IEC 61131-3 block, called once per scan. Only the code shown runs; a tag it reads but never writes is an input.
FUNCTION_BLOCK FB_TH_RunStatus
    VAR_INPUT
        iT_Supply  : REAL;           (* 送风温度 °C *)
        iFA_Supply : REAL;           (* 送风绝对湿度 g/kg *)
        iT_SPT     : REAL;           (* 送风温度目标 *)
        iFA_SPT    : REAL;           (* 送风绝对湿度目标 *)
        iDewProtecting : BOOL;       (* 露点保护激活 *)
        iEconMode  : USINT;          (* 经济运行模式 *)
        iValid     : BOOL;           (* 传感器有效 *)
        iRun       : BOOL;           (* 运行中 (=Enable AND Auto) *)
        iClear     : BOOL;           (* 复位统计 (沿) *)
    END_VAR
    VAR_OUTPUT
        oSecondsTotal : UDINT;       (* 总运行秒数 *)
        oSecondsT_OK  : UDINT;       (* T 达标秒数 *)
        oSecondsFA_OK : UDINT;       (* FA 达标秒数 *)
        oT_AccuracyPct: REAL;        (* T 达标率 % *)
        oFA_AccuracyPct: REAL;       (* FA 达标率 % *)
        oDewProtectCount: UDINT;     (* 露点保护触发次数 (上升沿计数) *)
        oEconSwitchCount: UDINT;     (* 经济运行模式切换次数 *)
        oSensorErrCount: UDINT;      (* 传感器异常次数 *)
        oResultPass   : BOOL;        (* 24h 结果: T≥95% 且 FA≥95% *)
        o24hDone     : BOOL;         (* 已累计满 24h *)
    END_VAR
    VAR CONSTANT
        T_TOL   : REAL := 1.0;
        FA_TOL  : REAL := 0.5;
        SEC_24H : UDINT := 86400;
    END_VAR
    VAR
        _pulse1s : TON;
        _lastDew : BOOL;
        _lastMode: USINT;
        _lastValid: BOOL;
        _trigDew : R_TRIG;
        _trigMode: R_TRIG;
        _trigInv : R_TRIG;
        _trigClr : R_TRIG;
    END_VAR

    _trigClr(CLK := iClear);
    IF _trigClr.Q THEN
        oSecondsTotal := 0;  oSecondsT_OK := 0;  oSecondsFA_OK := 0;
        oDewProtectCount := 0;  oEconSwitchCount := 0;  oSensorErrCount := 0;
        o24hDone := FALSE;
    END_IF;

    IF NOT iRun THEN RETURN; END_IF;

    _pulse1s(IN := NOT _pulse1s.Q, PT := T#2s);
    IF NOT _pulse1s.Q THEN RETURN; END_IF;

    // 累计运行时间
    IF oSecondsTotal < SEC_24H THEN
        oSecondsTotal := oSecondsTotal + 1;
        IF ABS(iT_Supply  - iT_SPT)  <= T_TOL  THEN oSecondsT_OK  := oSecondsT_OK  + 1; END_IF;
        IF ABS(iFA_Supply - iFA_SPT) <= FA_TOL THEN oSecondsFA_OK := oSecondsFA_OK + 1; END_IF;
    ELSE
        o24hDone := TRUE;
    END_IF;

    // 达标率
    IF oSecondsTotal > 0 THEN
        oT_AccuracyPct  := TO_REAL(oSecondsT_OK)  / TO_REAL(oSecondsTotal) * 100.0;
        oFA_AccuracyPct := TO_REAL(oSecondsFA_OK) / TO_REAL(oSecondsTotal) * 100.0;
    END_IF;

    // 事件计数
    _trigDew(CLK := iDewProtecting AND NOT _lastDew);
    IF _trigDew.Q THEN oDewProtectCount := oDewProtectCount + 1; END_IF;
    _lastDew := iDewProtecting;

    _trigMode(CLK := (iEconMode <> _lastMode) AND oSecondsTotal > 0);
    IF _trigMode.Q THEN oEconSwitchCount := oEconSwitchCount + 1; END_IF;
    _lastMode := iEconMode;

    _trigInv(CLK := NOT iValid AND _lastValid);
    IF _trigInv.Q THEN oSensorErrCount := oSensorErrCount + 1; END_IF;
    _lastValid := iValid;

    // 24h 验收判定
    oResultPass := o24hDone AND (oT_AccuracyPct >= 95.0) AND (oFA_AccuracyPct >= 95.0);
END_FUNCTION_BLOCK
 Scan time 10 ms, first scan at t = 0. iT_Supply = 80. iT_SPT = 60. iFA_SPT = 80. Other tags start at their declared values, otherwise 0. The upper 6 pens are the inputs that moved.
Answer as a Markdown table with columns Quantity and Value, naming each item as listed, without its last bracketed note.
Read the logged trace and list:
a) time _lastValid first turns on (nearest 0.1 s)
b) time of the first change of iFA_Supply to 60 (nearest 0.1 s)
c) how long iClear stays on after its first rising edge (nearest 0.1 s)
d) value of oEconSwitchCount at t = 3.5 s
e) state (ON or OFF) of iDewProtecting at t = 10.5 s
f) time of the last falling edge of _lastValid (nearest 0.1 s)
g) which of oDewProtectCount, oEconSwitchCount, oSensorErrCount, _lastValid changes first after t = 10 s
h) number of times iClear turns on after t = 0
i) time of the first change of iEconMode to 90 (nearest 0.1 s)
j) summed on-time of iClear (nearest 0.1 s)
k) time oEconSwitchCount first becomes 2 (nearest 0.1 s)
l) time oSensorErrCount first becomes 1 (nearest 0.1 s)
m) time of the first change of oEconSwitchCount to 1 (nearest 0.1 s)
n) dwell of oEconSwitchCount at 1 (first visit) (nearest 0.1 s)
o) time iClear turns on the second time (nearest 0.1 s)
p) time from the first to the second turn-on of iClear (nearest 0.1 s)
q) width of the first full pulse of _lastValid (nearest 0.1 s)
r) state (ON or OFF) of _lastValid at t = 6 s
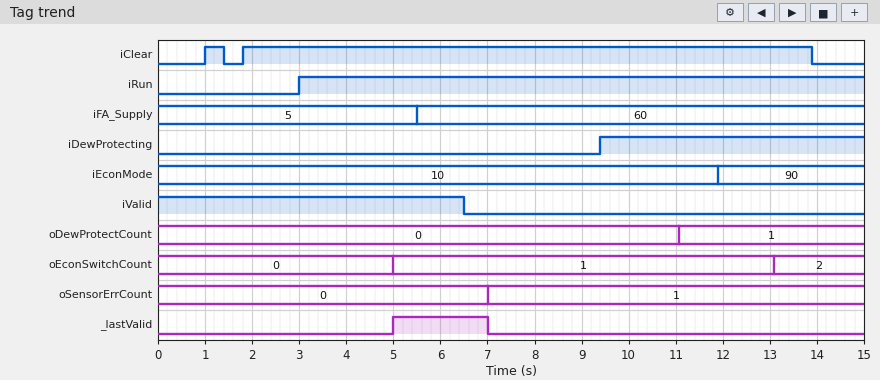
| Quantity | Value |
|---|---|
| time _lastValid first turns on | 5.0 s |
| time of the first change of iFA_Supply to 60 | 5.5 s |
| how long iClear stays on after its first rising edge | 0.4 s |
| value of oEconSwitchCount at t = 3.5 s | 0 |
| state (ON or OFF) of iDewProtecting at t = 10.5 s | ON |
| time of the last falling edge of _lastValid | 7.0 s |
| which of oDewProtectCount, oEconSwitchCount, oSensorErrCount, _lastValid changes first after t = 10 s | oDewProtectCount |
| number of times iClear turns on after t = 0 | 2 |
| time of the first change of iEconMode to 90 | 11.9 s |
| summed on-time of iClear | 12.5 s |
| time oEconSwitchCount first becomes 2 | 13.1 s |
| time oSensorErrCount first becomes 1 | 7.0 s |
| time of the first change of oEconSwitchCount to 1 | 5.0 s |
| dwell of oEconSwitchCount at 1 (first visit) | 8.1 s |
| time iClear turns on the second time | 1.8 s |
| time from the first to the second turn-on of iClear | 0.8 s |
| width of the first full pulse of _lastValid | 2.0 s |
| state (ON or OFF) of _lastValid at t = 6 s | ON |
